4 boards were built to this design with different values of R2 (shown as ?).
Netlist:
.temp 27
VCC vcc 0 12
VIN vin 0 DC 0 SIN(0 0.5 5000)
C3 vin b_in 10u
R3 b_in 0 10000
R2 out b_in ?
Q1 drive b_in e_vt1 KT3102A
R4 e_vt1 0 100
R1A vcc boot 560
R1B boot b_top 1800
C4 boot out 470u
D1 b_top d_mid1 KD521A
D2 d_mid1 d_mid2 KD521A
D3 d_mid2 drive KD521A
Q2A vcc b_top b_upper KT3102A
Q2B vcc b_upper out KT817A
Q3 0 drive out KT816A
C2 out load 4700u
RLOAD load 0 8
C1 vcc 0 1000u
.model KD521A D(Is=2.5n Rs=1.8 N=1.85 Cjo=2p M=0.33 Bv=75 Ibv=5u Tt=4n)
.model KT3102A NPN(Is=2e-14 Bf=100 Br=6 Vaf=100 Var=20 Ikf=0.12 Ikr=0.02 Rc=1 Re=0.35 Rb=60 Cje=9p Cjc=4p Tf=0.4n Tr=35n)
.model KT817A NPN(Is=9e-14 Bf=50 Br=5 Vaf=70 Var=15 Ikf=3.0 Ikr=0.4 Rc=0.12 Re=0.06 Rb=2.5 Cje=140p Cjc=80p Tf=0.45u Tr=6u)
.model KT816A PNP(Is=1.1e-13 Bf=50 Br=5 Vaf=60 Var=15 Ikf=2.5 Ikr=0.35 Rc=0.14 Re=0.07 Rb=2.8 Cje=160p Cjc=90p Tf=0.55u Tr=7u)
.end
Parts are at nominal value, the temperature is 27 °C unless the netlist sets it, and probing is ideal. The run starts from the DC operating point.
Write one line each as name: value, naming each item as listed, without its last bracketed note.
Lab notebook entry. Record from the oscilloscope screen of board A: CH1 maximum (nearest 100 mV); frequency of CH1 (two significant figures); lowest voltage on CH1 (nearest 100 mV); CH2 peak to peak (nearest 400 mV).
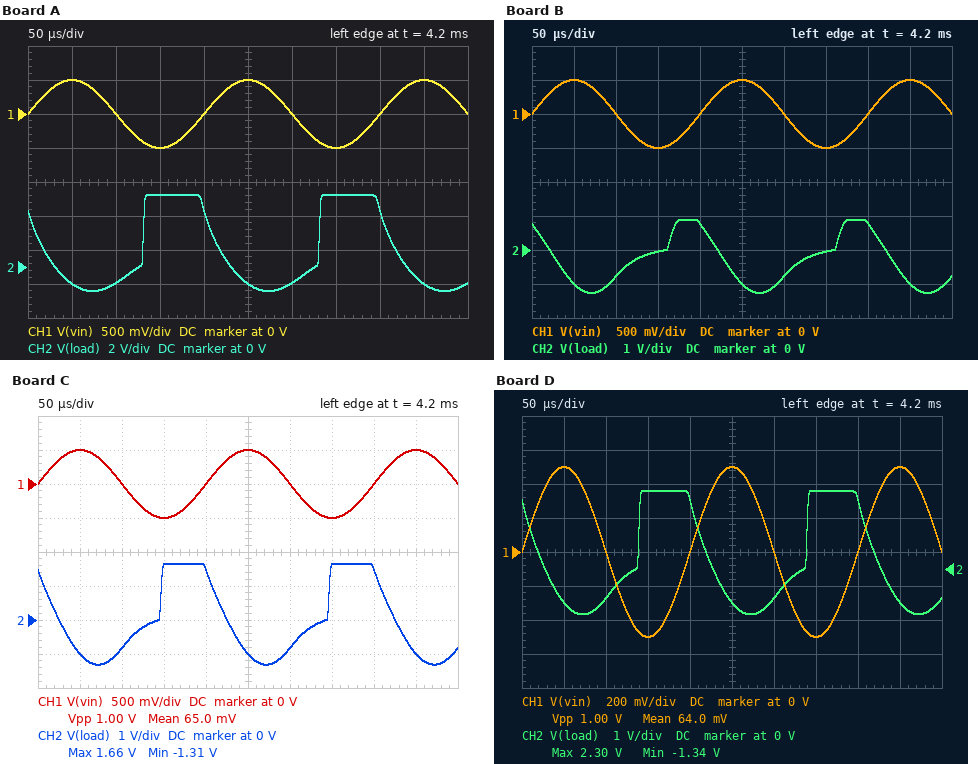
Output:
CH1 maximum: 500 mV
frequency of CH1: 5.0 kHz
lowest voltage on CH1: -500 mV
CH2 peak to peak: 5.6 V
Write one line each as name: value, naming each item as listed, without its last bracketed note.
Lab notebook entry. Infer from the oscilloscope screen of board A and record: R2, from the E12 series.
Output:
R2, from the E12 series: 56 kΩ
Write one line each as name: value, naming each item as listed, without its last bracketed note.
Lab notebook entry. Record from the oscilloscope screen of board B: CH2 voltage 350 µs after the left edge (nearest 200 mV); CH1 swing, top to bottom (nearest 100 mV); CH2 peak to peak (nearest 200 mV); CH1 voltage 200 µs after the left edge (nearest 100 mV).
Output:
CH2 voltage 350 µs after the left edge: 0 V
CH1 swing, top to bottom: 1.0 V
CH2 peak to peak: 2.2 V
CH1 voltage 200 µs after the left edge: 0 V
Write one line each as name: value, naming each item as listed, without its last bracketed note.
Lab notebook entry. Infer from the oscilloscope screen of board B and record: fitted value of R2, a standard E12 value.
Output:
fitted value of R2, a standard E12 value: 150 kΩ
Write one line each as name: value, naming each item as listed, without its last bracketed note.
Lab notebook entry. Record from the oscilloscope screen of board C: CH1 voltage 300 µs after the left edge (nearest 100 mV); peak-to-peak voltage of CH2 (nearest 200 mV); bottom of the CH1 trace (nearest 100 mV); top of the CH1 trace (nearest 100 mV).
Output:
CH1 voltage 300 µs after the left edge: 0 V
peak-to-peak voltage of CH2: 3.0 V
bottom of the CH1 trace: -500 mV
top of the CH1 trace: 500 mV
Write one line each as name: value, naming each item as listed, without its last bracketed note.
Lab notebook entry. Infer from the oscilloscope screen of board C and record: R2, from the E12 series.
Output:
R2, from the E12 series: 120 kΩ
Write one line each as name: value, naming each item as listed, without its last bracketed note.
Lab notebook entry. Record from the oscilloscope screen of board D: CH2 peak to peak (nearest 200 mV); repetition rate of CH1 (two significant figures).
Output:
CH2 peak to peak: 3.6 V
repetition rate of CH1: 5.0 kHz
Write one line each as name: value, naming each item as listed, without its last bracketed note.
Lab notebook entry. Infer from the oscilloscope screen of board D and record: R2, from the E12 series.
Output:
R2, from the E12 series: 100 kΩ
